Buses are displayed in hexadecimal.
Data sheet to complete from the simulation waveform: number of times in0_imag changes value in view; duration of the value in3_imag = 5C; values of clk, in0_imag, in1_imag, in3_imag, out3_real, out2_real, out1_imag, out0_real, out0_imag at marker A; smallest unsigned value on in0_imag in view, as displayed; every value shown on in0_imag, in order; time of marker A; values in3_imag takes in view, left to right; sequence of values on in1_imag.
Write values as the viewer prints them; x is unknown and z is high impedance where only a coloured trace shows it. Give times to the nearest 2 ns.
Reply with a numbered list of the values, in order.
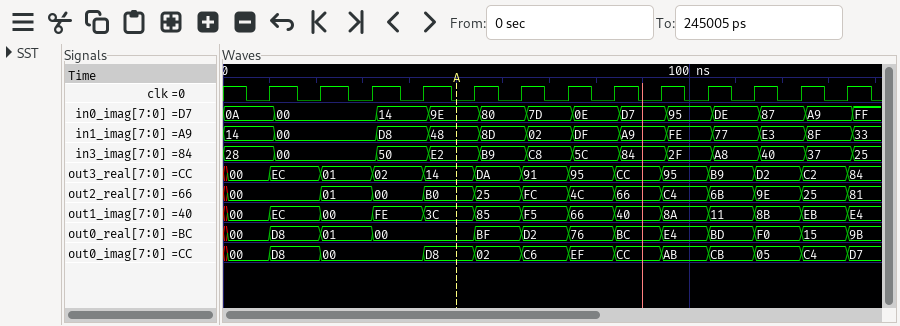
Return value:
1. 12
2. 10 ns
3. clk=0, in0_imag=9E, in1_imag=48, in3_imag=E2, out3_real=14, out2_real=B0, out1_imag=3C, out0_real=00, out0_imag=D8
4. 00
5. 0A, 00, 14, 9E, 80, 7D, 0E, D7, 95, DE, 87, A9, FF
6. 50 ns
7. 28, 00, 50, E2, B9, C8, 5C, 84, 2F, A8, 40, 37, 25
8. 14, 00, D8, 48, 8D, 02, DF, A9, FE, 77, E3, 8F, 33
